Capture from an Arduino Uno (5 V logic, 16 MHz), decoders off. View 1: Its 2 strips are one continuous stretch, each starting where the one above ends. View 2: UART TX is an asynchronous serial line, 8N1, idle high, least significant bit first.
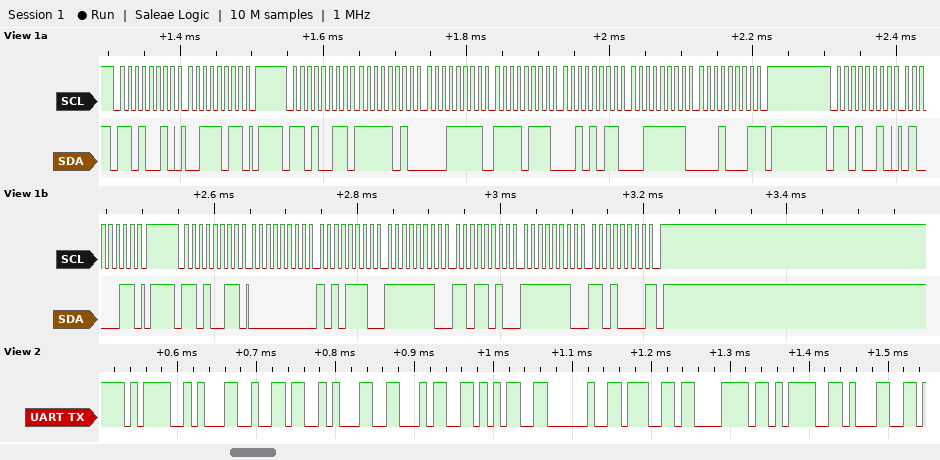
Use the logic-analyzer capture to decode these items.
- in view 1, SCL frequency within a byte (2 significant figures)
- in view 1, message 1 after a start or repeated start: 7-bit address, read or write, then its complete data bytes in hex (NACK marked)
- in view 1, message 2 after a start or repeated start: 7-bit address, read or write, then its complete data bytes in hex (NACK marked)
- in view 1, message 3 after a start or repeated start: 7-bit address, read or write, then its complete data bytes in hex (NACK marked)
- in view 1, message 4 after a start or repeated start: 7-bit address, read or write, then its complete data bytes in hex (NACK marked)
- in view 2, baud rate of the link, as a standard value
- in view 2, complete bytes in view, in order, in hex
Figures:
100 kHz
0x69 write: 3B
0x69 read: FA 1F F7 2B 3F 11 NACK
0x69 write: 43
0x69 read: 00 AE FE DA FE D0 NACK
115200 baud
3D 31 36 31 34 35 20 67 78 3D 31
